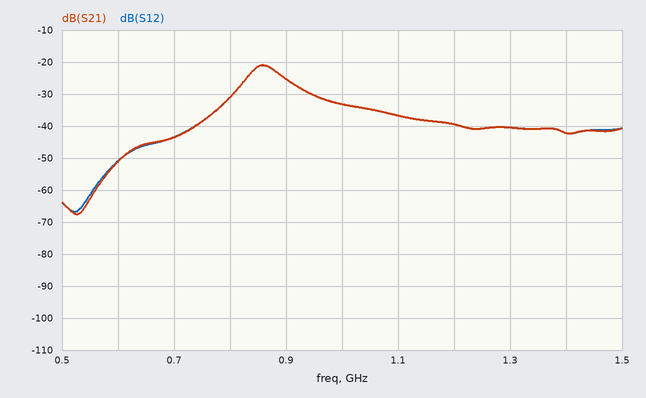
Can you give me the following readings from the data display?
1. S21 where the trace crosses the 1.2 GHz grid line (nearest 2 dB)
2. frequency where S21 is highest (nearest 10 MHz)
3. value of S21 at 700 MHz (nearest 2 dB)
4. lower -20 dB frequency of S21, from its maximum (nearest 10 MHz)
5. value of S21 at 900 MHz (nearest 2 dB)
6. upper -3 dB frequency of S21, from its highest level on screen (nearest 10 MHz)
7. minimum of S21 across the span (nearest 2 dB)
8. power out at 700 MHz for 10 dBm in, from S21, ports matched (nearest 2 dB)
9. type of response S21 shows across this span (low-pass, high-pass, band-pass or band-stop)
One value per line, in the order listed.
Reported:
-40 dB
860 MHz
-44 dB
730 MHz
-26 dB
890 MHz
-68 dB
-34 dBm
band-pass
